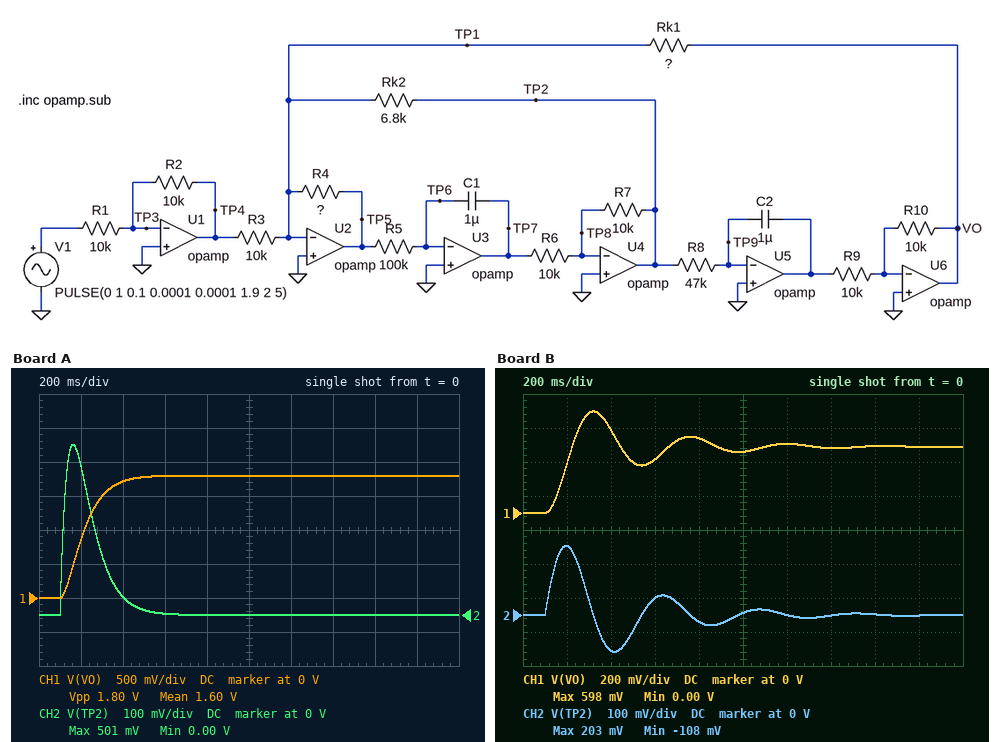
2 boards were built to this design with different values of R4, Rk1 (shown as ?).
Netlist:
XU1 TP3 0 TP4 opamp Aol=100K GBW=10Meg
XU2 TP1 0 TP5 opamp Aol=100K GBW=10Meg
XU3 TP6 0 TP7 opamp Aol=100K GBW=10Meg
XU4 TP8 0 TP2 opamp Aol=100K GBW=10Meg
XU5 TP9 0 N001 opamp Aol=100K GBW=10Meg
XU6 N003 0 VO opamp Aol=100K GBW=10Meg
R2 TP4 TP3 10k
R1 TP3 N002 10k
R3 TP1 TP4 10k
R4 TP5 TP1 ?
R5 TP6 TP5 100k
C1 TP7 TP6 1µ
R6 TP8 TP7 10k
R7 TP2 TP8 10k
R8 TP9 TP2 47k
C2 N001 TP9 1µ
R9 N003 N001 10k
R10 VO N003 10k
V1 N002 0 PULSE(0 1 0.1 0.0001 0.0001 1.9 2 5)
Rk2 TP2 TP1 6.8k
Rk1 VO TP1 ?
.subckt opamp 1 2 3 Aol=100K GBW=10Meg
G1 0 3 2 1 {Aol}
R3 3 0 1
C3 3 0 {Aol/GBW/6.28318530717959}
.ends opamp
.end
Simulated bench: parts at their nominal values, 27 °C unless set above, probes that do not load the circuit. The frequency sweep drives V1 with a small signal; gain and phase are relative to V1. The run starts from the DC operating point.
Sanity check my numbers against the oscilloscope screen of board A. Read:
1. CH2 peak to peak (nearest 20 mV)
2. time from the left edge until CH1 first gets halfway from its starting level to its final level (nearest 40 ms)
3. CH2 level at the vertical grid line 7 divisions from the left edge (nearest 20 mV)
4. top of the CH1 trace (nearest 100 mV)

500 mV
200 ms
0 V
1.8 V
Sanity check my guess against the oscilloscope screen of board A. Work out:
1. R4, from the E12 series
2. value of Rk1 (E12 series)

22 kΩ
18 kΩ
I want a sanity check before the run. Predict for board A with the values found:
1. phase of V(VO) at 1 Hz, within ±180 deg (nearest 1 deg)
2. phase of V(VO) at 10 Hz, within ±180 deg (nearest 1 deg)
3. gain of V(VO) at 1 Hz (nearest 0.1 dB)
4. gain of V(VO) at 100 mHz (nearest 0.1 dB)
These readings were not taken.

-43 deg
-151 deg
3.9 dB
5.1 dB
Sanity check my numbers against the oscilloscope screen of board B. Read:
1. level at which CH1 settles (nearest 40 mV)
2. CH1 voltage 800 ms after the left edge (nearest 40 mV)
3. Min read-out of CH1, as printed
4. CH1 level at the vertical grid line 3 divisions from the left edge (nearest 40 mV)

400 mV
440 mV
0.00 V
320 mV
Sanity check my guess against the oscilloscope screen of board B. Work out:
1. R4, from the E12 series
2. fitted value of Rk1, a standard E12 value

3.9 kΩ
3.9 kΩ
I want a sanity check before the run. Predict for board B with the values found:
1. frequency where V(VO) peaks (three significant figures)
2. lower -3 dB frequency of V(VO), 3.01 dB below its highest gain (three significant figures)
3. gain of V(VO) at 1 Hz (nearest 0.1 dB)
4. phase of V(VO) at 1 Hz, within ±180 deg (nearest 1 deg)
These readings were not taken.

2.23 Hz
1.70 Hz
-6.6 dB
-12 deg
